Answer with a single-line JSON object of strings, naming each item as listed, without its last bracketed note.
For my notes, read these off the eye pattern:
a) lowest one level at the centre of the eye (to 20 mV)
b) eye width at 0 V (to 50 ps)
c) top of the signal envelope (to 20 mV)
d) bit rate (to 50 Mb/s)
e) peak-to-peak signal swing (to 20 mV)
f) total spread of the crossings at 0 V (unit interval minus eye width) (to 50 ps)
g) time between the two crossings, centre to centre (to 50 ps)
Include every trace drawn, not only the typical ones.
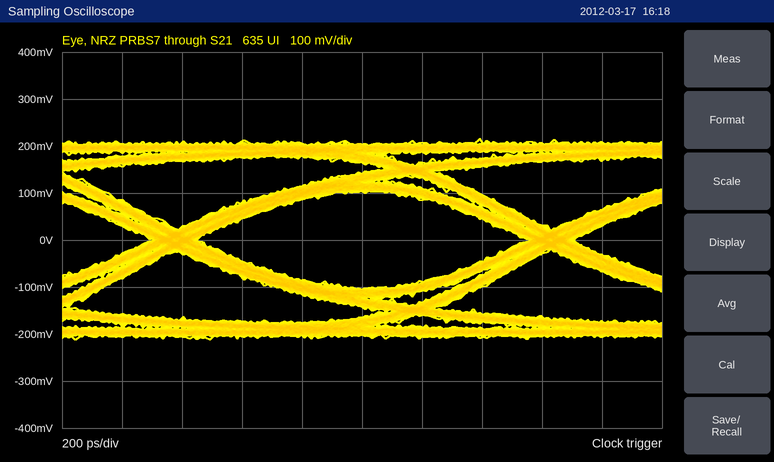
{"lowest one level at the centre of the eye": "100 mV", "eye width at 0 V": "1.10 ns", "top of the signal envelope": "220 mV", "bit rate": "800 Mb/s", "peak-to-peak signal swing": "420 mV", "total spread of the crossings at 0 V (unit interval minus eye width)": "150 ps", "time between the two crossings, centre to centre": "1.25 ns"}
